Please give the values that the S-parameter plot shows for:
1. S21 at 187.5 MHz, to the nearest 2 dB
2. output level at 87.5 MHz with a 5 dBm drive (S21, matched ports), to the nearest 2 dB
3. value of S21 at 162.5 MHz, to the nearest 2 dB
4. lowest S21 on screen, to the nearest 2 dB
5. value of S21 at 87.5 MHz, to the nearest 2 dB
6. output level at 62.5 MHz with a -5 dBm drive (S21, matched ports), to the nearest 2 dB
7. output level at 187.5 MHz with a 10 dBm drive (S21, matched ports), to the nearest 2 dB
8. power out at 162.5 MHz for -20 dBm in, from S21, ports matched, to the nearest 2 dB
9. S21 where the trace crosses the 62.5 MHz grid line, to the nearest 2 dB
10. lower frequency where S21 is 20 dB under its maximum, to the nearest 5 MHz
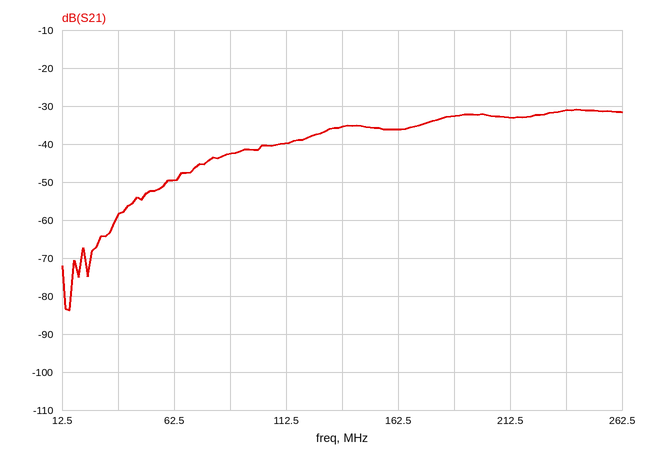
-32 dB
-38 dBm
-36 dB
-84 dB
-42 dB
-54 dBm
-22 dBm
-56 dBm
-50 dB
60 MHz
